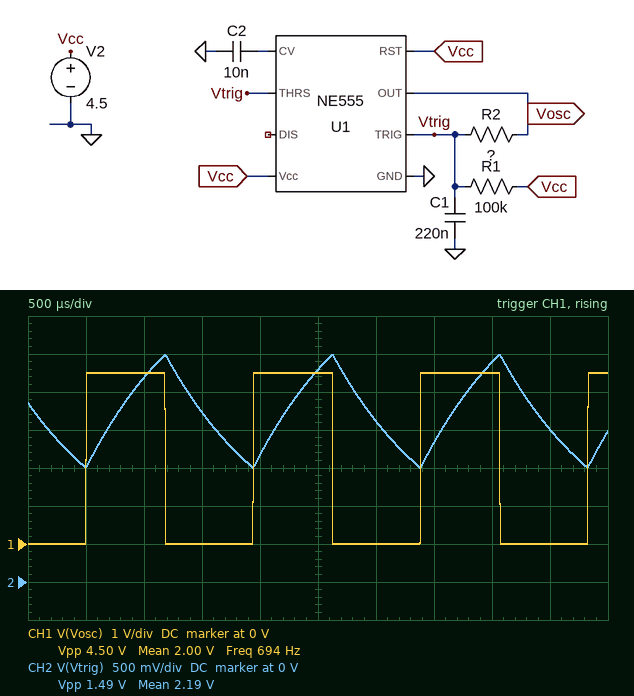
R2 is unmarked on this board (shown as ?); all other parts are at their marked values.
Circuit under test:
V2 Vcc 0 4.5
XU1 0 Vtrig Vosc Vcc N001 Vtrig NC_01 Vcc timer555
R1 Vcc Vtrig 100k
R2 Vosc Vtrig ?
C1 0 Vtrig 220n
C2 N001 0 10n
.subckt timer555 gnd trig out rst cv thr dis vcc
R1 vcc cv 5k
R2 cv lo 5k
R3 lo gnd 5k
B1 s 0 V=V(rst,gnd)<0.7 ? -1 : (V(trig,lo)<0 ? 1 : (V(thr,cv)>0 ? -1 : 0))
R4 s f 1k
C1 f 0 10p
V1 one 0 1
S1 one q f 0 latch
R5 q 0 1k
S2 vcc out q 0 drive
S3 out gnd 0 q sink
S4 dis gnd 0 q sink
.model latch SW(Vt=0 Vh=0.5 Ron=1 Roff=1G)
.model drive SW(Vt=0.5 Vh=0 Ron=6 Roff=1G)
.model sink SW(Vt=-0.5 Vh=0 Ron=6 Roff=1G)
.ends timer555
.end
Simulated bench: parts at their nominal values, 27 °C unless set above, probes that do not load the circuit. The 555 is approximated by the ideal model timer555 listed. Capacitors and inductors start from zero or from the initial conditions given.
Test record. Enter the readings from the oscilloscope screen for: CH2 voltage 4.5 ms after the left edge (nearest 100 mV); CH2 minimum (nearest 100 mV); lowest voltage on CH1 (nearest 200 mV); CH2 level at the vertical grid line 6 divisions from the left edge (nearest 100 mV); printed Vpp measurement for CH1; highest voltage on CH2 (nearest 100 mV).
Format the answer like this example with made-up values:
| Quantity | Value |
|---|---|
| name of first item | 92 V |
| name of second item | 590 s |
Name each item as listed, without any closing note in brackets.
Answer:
| Quantity | Value |
|---|---|
| CH2 voltage 4.5 ms after the left edge | 2.0 V |
| CH2 minimum | 1.5 V |
| lowest voltage on CH1 | 0 V |
| CH2 level at the vertical grid line 6 divisions from the left edge | 2.1 V |
| printed Vpp measurement for CH1 | 4.50 V |
| highest voltage on CH2 | 3.0 V |
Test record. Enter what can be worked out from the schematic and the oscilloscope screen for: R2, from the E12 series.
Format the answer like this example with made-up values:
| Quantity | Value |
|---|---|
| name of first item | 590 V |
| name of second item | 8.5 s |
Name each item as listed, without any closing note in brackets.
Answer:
| Quantity | Value |
|---|---|
| R2, from the E12 series | 4.7 kΩ |
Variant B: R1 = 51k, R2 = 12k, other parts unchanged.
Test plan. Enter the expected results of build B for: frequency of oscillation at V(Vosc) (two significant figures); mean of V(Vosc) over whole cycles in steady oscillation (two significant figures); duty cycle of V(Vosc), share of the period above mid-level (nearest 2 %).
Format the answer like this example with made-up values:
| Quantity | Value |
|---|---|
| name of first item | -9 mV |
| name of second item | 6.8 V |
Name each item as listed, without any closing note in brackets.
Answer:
| Quantity | Value |
|---|---|
| frequency of oscillation at V(Vosc) | 250 Hz |
| mean of V(Vosc) over whole cycles in steady oscillation | 1.6 V |
| duty cycle of V(Vosc), share of the period above mid-level | 36 % |
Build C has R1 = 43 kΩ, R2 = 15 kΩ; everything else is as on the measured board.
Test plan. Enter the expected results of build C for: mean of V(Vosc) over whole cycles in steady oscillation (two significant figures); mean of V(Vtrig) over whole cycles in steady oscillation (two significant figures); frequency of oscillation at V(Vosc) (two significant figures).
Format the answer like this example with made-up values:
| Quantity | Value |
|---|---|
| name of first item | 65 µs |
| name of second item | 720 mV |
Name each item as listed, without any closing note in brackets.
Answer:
| Quantity | Value |
|---|---|
| mean of V(Vosc) over whole cycles in steady oscillation | 1.3 V |
| mean of V(Vtrig) over whole cycles in steady oscillation | 2.1 V |
| frequency of oscillation at V(Vosc) | 170 Hz |
